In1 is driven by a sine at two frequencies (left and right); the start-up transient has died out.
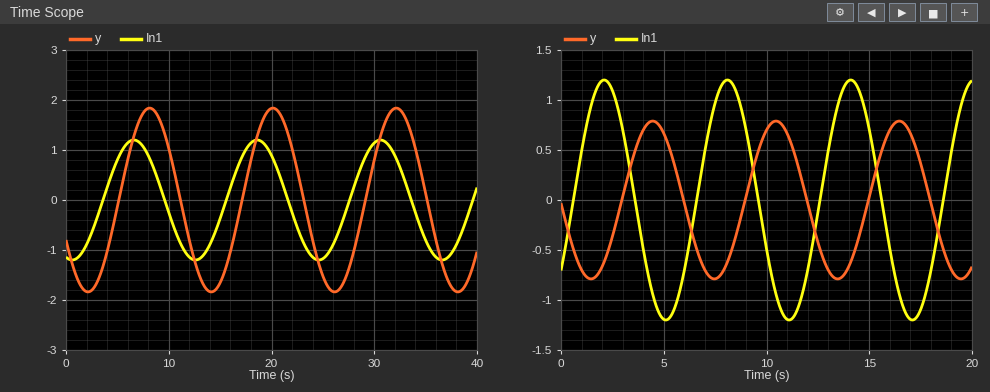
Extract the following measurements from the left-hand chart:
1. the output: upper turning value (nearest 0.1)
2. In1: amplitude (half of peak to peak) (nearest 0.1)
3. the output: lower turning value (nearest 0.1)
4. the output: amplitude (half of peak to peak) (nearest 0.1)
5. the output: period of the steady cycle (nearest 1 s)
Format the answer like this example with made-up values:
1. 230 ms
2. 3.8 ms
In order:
1. 1.8
2. 1.2
3. -1.8
4. 1.8
5. 12 s
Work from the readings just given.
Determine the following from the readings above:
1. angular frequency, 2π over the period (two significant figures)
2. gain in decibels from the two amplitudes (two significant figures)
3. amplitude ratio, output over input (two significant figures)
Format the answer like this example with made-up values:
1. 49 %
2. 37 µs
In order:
1. 0.52 rad/s
2. 3.5 dB
3. 1.5
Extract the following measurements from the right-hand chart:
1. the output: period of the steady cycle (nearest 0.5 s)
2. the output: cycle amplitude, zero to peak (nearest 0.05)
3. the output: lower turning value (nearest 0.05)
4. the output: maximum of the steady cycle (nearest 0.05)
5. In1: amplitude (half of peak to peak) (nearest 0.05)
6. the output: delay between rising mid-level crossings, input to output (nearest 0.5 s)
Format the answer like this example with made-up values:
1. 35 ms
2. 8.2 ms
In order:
1. 6.0 s
2. 0.80
3. -0.80
4. 0.80
5. 1.20
6. 2.5 s
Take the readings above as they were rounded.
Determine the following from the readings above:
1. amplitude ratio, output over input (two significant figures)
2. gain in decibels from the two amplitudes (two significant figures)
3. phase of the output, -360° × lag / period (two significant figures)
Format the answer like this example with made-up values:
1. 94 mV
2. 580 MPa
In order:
1. 0.67
2. -3.5 dB
3. -150°
